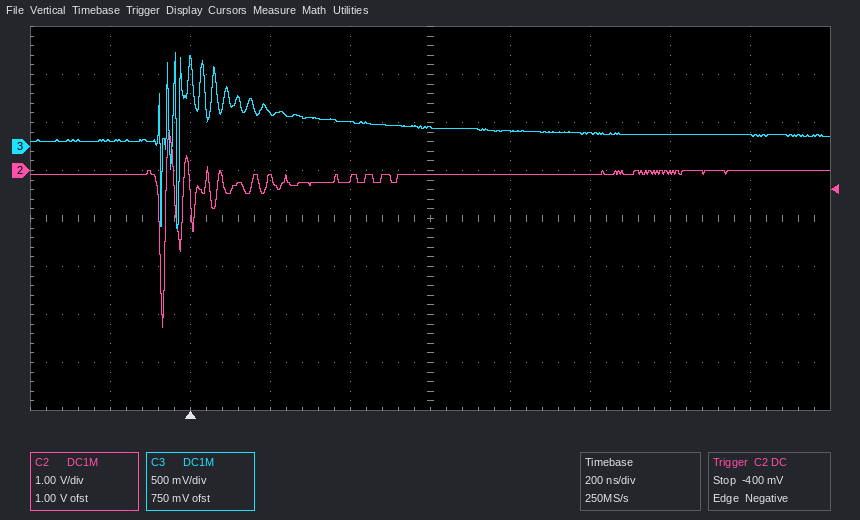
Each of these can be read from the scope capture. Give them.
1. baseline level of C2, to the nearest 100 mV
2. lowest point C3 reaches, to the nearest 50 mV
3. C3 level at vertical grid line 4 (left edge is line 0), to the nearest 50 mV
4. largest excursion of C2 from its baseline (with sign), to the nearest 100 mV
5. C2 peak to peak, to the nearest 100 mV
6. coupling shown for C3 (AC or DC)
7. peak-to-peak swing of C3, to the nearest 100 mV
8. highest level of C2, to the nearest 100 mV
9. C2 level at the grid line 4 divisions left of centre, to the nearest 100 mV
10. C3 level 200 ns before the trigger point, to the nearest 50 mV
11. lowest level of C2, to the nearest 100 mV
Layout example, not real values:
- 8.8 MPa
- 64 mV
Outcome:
- -100 mV
- -850 mV
- 250 mV
- -3.2 V
- 4.1 V
- DC
- 1.80 V
- 800 mV
- -100 mV
- 50 mV
- -3.3 V
